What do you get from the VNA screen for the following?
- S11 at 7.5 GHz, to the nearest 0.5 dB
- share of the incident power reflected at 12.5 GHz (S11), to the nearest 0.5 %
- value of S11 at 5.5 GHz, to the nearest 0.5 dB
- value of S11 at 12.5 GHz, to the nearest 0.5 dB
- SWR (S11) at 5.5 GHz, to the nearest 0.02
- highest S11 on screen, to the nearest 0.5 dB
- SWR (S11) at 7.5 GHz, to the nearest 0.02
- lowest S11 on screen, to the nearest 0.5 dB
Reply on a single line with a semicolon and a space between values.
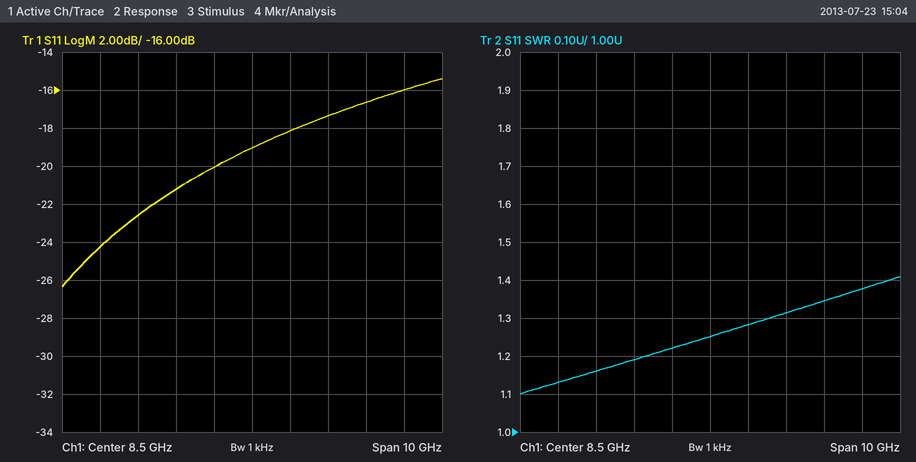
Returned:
-20.0 dB; 2.5 %; -22.5 dB; -16.0 dB; 1.16; -15.5 dB; 1.22; -26.5 dB
